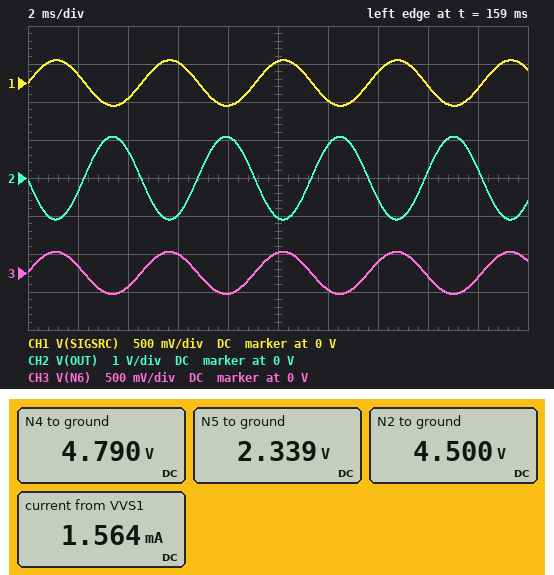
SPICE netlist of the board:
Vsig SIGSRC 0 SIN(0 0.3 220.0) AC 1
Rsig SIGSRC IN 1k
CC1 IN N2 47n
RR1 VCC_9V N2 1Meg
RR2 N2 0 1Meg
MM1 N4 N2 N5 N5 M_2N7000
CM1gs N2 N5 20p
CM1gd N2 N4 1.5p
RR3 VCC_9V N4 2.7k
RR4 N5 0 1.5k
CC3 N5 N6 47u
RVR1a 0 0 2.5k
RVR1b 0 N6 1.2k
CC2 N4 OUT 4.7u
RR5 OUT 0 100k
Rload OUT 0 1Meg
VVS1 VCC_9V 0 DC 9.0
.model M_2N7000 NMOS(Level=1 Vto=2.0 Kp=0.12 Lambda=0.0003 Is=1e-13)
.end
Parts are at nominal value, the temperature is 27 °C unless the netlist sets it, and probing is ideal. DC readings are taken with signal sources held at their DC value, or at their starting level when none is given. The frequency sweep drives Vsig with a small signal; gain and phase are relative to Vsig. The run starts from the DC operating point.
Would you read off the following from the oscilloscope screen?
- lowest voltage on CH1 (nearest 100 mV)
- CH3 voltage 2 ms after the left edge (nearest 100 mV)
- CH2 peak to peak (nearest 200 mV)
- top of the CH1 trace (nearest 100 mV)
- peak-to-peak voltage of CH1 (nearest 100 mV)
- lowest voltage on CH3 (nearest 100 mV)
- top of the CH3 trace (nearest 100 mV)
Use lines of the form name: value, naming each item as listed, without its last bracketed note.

lowest voltage on CH1: -300 mV
CH3 voltage 2 ms after the left edge: 100 mV
CH2 peak to peak: 2.2 V
top of the CH1 trace: 300 mV
peak-to-peak voltage of CH1: 600 mV
lowest voltage on CH3: -300 mV
top of the CH3 trace: 300 mV
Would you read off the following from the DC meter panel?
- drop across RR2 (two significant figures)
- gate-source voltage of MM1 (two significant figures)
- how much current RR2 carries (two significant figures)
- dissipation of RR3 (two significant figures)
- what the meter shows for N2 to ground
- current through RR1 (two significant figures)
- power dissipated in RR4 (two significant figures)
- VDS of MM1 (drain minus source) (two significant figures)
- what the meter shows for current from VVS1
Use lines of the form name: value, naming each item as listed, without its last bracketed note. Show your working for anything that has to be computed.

drop across RR2: 4.5 V = 4.5 V
gate-source voltage of MM1: 4.5 V - 2.339 V = 2.2 V
how much current RR2 carries: (4.5 V) / 1 MΩ = 4.5 µA
dissipation of RR3: (9 V - 4.79 V)^2 / 2.7 kΩ = 6.6 mW
what the meter shows for N2 to ground: 4.500 V
current through RR1: (9 V - 4.5 V) / 1 MΩ = 4.5 µA
power dissipated in RR4: (2.339 V)^2 / 1.5 kΩ = 3.6 mW
VDS of MM1 (drain minus source): 4.79 V - 2.339 V = 2.5 V
what the meter shows for current from VVS1: 1.564 mA
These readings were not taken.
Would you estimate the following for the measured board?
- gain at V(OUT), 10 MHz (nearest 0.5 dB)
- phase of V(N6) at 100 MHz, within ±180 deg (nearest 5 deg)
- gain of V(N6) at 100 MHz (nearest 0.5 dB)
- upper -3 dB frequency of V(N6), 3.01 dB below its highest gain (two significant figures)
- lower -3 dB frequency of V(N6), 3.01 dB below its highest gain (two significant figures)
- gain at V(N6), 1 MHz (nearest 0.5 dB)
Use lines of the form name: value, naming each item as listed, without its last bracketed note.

gain at V(OUT), 10 MHz: 9.0 dB
phase of V(N6) at 100 MHz, within ±180 deg: -10 deg
gain of V(N6) at 100 MHz: -9.5 dB
upper -3 dB frequency of V(N6), 3.01 dB below its highest gain: 14 MHz
lower -3 dB frequency of V(N6), 3.01 dB below its highest gain: 7.7 Hz
gain at V(N6), 1 MHz: -0.5 dB
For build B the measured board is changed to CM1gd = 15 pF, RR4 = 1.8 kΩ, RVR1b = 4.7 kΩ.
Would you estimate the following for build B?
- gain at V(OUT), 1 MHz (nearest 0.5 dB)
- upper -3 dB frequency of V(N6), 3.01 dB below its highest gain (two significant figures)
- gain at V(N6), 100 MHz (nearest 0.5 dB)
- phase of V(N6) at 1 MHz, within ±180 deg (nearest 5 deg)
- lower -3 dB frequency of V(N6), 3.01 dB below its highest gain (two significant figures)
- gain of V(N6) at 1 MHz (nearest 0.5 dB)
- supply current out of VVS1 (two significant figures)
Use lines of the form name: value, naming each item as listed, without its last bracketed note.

gain at V(OUT), 1 MHz: 4.5 dB
upper -3 dB frequency of V(N6), 3.01 dB below its highest gain: 2.5 MHz
gain at V(N6), 100 MHz: -7.0 dB
phase of V(N6) at 1 MHz, within ±180 deg: -15 deg
lower -3 dB frequency of V(N6), 3.01 dB below its highest gain: 6.8 Hz
gain of V(N6) at 1 MHz: -1.0 dB
supply current out of VVS1: 1.3 mA
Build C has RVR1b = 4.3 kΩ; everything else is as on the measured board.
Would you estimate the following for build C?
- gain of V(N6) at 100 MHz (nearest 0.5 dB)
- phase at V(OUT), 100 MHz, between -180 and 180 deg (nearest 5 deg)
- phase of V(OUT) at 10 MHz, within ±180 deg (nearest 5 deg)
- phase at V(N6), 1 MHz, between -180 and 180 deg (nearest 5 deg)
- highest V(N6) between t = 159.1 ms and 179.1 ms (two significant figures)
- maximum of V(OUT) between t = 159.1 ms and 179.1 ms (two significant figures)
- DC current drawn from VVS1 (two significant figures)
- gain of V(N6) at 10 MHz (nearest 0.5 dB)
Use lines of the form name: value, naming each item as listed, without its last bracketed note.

gain of V(N6) at 100 MHz: -7.5 dB
phase at V(OUT), 100 MHz, between -180 and 180 deg: 35 deg
phase of V(OUT) at 10 MHz, within ±180 deg: 140 deg
phase at V(N6), 1 MHz, between -180 and 180 deg: 0 deg
highest V(N6) between t = 159.1 ms and 179.1 ms: 290 mV
maximum of V(OUT) between t = 159.1 ms and 179.1 ms: 670 mV
DC current drawn from VVS1: 1.6 mA
gain of V(N6) at 10 MHz: -1.5 dB
